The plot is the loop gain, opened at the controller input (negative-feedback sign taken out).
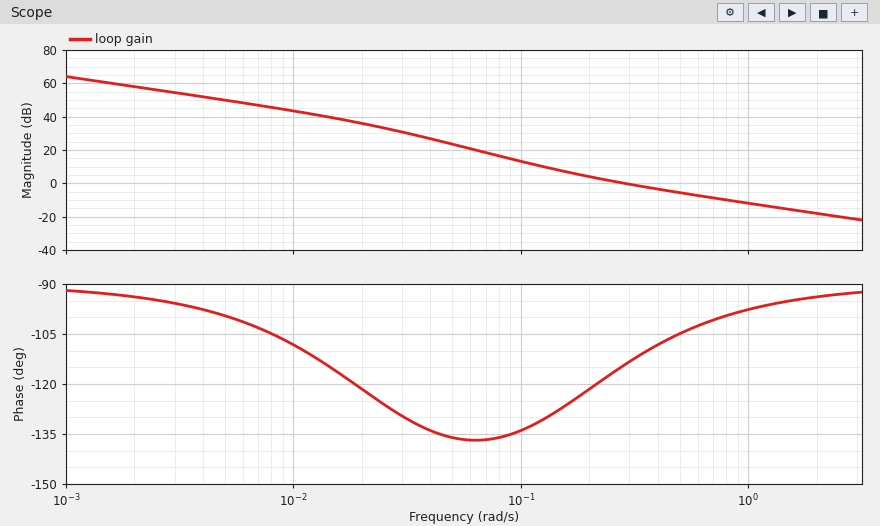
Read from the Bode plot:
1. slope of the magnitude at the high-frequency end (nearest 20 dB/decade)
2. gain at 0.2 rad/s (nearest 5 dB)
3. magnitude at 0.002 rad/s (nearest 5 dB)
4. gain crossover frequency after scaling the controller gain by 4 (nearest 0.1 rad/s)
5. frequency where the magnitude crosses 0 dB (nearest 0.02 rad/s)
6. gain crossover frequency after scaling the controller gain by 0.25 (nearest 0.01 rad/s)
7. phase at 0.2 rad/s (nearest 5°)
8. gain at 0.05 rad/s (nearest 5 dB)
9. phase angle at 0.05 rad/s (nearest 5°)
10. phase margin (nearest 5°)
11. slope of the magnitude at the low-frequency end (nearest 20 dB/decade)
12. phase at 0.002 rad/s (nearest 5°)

-20 dB/decade
5 dB
60 dB
1.0 rad/s
0.28 rad/s
0.11 rad/s
-120°
25 dB
-135°
65°
-20 dB/decade
-95°
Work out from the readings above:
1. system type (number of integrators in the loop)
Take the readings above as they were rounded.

1
